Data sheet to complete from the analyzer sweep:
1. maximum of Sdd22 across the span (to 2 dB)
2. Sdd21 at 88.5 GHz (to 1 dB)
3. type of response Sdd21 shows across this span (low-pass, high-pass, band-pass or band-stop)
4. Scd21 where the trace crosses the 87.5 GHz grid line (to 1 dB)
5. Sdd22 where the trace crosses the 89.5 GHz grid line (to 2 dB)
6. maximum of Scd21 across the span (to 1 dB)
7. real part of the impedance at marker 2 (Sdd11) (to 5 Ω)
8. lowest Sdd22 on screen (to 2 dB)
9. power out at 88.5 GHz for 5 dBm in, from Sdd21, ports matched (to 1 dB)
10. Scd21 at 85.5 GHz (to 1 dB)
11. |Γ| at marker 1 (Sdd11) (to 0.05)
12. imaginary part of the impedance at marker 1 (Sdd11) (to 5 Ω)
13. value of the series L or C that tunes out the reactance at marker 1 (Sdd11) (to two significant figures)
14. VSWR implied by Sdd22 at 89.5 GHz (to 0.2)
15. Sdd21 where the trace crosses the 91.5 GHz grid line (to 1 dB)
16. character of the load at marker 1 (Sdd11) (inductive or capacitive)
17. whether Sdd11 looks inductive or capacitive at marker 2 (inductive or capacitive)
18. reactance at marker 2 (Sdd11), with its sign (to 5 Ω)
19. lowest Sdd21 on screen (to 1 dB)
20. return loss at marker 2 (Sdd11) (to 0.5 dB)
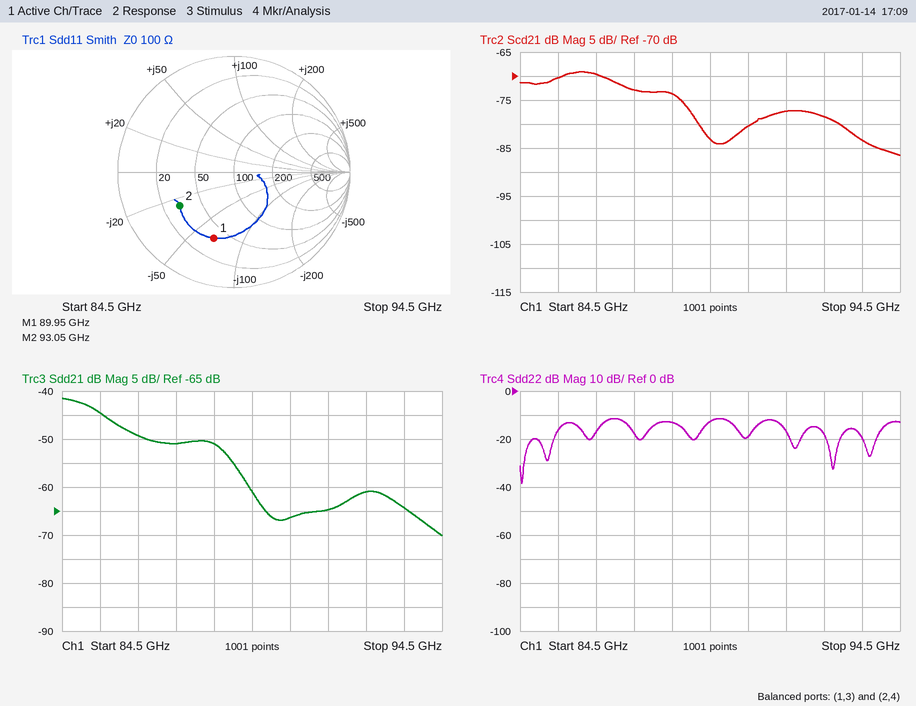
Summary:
-12 dB
-51 dB
low-pass
-73 dB
-12 dB
-69 dB
30 Ω
-38 dB
-46 dBm
-70 dB
0.60
-65 Ω
120 pH
1.6
-65 dB
capacitive
capacitive
-25 Ω
-70 dB
5.0 dB
